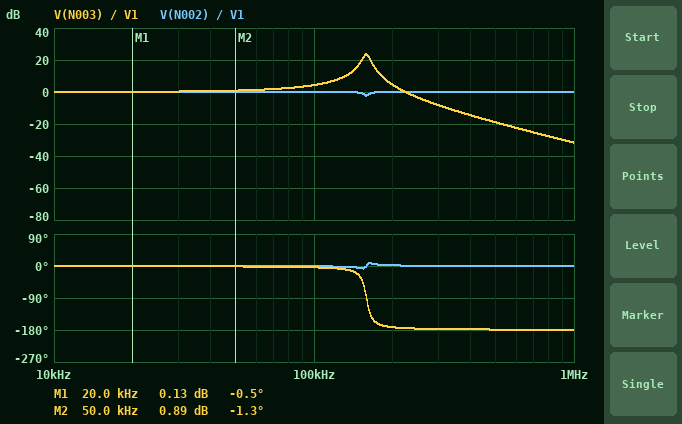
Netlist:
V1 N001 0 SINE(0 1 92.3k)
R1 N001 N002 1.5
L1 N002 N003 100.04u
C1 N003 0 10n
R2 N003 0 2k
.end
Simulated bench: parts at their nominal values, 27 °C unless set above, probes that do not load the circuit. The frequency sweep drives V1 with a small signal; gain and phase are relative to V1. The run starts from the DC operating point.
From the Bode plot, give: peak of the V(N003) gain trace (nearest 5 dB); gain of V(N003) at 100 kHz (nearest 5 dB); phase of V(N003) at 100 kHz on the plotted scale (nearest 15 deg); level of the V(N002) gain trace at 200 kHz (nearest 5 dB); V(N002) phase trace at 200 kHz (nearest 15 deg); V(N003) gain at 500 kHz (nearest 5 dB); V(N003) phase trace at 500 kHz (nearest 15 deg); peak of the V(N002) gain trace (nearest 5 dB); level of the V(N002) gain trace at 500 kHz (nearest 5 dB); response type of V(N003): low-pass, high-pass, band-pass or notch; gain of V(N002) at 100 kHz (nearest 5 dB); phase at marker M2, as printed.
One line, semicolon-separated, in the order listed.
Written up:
25 dB; 5 dB; 0 deg; 0 dB; 0 deg; -20 dB; -180 deg; 0 dB; 0 dB; band-pass; 0 dB; -1.3 deg
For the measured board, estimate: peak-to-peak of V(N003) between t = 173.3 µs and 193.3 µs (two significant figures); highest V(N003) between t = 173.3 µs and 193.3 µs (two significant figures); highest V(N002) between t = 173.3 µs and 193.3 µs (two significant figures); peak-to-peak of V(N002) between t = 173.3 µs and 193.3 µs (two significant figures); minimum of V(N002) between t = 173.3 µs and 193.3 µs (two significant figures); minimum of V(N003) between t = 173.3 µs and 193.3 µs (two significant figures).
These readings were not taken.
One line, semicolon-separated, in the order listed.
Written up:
3.0 V; 1.5 V; 1.0 V; 2.0 V; -1.0 V; -1.5 V
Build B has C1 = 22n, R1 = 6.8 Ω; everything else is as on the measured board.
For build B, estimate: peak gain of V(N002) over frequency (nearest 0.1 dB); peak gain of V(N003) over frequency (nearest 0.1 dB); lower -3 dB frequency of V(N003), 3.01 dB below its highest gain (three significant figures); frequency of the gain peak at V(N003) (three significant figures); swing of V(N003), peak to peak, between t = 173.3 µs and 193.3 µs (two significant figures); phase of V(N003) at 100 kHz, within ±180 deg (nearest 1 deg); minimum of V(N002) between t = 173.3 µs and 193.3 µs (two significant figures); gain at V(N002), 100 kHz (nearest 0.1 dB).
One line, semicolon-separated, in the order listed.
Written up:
0 dB; 17.4 dB; 99.5 kHz; 107 kHz; 7.0 V; -43 deg; -910 mV; -2.7 dB
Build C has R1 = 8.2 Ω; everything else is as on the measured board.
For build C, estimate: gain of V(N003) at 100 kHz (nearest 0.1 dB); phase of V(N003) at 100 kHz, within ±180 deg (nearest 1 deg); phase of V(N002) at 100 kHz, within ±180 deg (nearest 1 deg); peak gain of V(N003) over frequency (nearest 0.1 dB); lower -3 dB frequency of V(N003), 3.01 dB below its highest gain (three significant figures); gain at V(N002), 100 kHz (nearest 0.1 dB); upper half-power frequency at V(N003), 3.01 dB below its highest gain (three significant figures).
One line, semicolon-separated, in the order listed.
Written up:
4.2 dB; -8 deg; -5 deg; 17.6 dB; 148 kHz; -0.1 dB; 169 kHz
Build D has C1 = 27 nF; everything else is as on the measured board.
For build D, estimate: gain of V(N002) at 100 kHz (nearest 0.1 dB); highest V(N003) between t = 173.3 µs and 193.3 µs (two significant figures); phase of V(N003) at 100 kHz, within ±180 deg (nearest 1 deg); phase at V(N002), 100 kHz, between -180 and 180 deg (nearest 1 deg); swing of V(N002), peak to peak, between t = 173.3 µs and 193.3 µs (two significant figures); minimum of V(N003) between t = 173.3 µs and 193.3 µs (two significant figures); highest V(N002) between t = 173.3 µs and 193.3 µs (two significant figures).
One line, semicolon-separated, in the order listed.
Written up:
-1.5 dB; 9.3 V; -139 deg; 16 deg; 1.8 V; -9.2 V; 920 mV
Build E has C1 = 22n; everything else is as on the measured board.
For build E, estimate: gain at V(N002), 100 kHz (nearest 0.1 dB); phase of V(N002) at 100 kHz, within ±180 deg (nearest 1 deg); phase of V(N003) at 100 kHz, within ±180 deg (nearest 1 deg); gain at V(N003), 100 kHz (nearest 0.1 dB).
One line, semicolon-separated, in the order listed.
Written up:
-0.4 dB; -8 deg; -22 deg; 17.0 dB
